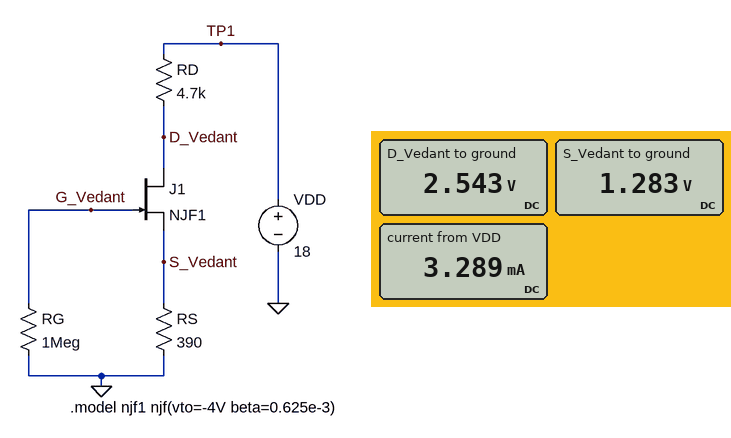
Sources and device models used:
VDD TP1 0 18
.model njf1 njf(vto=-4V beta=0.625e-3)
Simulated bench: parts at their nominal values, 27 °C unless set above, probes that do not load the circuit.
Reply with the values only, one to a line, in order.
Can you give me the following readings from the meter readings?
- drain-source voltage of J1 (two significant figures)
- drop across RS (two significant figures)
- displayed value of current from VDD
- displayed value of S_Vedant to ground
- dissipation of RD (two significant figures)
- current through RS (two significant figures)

1.3 V
1.3 V
3.289 mA
1.283 V
51 mW
3.3 mA
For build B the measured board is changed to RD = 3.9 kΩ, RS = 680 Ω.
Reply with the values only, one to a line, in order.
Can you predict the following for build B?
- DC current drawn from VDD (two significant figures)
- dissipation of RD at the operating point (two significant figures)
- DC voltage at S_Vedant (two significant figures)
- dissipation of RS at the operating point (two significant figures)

2.8 mA
30 mW
1.9 V
5.3 mW
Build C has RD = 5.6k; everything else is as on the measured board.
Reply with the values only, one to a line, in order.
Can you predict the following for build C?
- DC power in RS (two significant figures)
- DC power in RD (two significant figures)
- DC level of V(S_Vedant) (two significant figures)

3.2 mW
45 mW
1.1 V
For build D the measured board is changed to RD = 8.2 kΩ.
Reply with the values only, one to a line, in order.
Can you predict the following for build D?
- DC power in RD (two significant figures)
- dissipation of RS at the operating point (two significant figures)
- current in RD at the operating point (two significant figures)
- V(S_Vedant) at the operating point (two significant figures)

34 mW
1.6 mW
2.0 mA
790 mV
